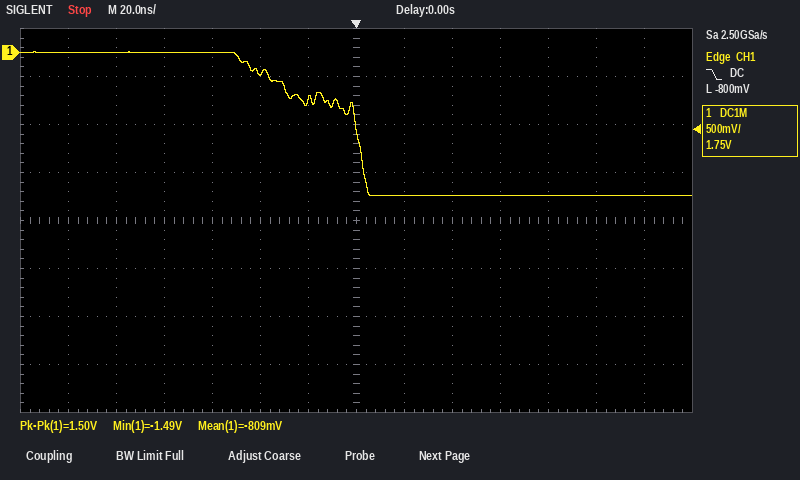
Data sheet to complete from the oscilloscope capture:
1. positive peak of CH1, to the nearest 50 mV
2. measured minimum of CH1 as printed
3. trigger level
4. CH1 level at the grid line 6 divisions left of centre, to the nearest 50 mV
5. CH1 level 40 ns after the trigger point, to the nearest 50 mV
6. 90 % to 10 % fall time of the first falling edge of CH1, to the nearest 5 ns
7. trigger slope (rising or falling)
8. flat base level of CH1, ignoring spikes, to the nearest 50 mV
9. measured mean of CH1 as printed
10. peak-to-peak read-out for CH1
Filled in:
0 mV
-1.49 V
-800 mV
0 mV
-1.50 V
50 ns
falling
-1.50 V
-809 mV
1.50 V
